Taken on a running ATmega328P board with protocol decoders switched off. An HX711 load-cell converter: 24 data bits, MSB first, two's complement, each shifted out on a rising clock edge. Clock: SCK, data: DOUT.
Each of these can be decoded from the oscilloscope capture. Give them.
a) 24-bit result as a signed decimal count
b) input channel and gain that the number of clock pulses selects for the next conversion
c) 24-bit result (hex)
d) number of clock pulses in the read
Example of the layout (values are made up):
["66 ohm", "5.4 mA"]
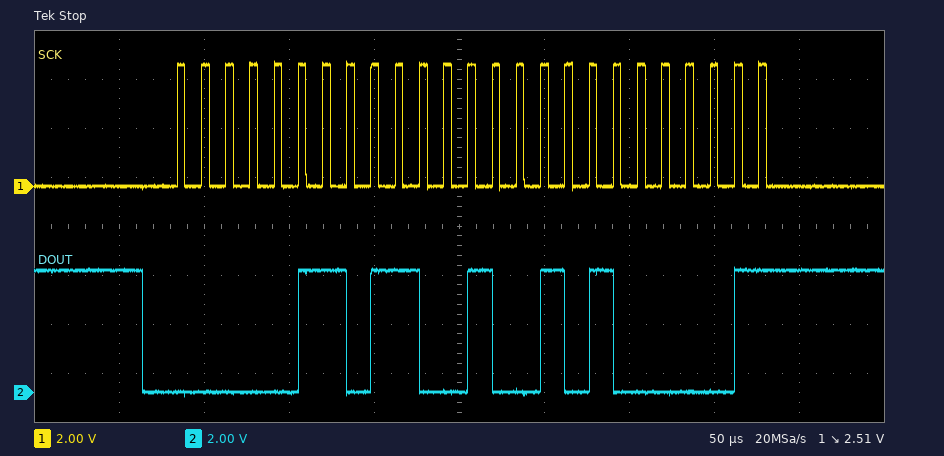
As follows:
["444737", "channel A, gain 128", "0x06C941", "25"]
